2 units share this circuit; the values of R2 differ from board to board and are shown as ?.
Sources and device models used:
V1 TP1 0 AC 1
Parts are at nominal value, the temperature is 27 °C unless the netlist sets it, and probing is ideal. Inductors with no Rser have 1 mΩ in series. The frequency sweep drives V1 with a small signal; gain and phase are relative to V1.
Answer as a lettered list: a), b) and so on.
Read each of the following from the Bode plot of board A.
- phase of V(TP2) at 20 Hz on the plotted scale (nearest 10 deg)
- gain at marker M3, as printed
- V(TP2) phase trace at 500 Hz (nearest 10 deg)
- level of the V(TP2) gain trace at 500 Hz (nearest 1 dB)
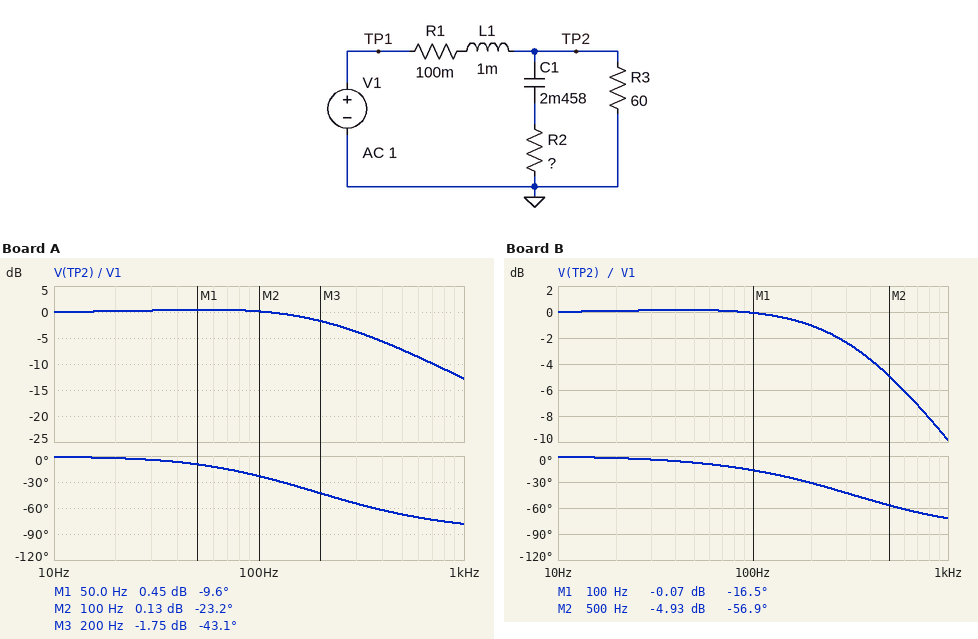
a) 0 deg
b) -1.75 dB
c) -70 deg
d) -7 dB
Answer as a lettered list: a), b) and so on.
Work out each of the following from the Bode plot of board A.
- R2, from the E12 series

a) 1.5 Ω
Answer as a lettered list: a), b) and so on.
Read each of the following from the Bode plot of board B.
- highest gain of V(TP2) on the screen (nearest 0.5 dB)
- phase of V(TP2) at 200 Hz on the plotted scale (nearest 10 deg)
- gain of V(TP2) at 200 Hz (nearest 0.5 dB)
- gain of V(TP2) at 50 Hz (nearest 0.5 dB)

a) 0 dB
b) -30 deg
c) -1.0 dB
d) 0 dB
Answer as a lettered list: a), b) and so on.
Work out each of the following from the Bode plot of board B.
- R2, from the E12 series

a) 2.2 Ω
